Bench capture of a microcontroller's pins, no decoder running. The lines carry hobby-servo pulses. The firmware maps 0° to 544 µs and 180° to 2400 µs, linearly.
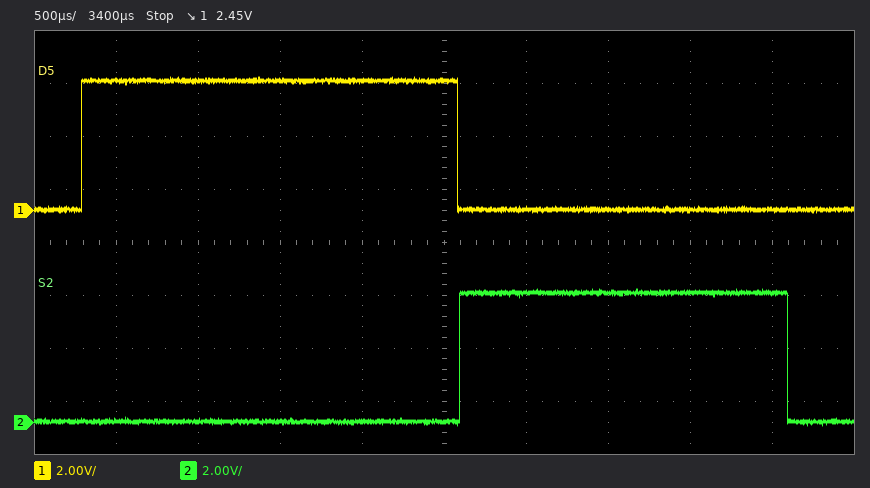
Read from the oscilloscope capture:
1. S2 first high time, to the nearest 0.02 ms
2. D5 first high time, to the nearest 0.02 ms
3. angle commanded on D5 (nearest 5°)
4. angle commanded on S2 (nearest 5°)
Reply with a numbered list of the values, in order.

1. 2.00 ms
2. 2.30 ms
3. 170°
4. 140°
